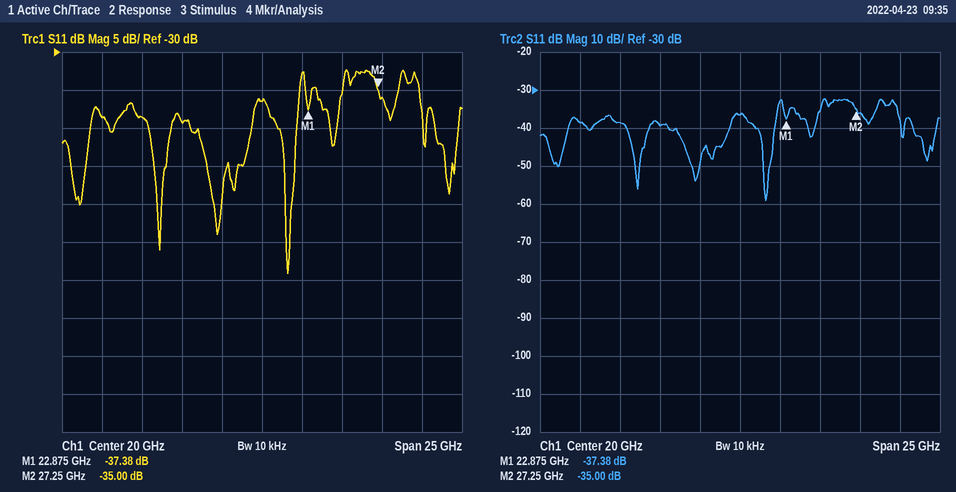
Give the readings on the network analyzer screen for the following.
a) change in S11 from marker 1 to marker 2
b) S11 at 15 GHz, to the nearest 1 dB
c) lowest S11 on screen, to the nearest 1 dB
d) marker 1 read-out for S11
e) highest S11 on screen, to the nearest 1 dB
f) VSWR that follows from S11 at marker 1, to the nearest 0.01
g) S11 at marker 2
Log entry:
2.38 dB
-39 dB
-59 dB
-37.38 dB
-32 dB
1.03
-35.00 dB
